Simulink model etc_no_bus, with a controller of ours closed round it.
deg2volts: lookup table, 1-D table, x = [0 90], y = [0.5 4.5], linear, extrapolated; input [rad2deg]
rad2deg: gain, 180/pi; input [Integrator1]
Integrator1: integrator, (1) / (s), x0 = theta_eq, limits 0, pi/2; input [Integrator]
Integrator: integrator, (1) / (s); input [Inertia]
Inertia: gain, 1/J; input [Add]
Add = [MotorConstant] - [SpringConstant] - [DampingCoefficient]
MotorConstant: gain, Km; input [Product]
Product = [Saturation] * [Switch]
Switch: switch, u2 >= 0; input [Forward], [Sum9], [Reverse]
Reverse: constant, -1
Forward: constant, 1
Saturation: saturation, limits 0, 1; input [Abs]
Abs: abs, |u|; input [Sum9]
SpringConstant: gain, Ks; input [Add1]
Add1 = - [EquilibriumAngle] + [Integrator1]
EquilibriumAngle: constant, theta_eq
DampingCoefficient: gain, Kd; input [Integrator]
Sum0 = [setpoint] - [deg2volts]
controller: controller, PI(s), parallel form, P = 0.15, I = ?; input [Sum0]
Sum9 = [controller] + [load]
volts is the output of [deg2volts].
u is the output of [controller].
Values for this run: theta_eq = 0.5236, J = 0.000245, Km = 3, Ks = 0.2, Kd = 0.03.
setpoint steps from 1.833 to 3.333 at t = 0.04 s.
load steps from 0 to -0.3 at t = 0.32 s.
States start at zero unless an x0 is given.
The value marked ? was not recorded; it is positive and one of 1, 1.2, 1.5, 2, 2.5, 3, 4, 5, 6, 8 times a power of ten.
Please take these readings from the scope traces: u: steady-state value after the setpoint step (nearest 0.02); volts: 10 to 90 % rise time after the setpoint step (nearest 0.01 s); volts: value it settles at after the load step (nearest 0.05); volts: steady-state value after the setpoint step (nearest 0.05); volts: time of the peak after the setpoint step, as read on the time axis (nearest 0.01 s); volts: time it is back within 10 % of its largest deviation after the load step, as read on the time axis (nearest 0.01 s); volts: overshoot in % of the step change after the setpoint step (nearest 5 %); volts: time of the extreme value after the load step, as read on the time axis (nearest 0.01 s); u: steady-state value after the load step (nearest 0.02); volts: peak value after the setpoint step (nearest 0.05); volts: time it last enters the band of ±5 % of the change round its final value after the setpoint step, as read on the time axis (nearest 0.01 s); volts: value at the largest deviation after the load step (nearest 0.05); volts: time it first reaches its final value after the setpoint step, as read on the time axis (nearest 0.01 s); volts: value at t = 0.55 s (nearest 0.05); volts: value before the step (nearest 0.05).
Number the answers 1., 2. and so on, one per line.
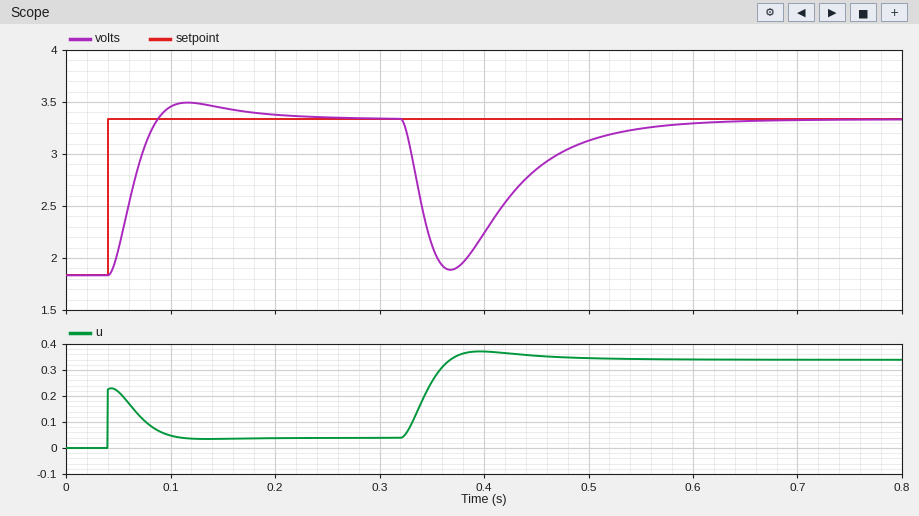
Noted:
1. 0.04
2. 0.03 s
3. 3.35
4. 3.35
5. 0.12 s
6. 0.52 s
7. 10 %
8. 0.37 s
9. 0.34
10. 3.50
11. 0.17 s
12. 1.90
13. 0.09 s
14. 3.25
15. 1.85
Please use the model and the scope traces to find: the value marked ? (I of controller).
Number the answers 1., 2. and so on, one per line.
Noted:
1. 2
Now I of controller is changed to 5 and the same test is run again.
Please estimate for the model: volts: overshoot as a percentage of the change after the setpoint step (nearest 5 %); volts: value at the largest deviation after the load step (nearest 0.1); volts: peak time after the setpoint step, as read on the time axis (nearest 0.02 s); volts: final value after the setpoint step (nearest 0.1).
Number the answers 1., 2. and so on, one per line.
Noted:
1. 35 %
2. 2.1
3. 0.10 s
4. 3.3
